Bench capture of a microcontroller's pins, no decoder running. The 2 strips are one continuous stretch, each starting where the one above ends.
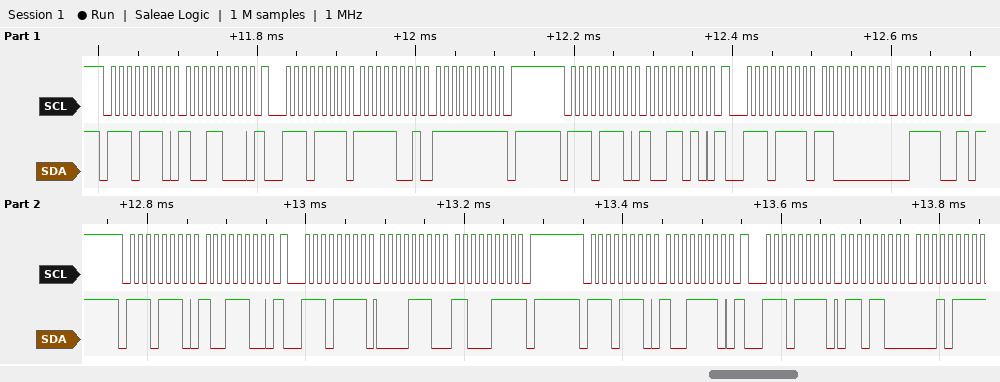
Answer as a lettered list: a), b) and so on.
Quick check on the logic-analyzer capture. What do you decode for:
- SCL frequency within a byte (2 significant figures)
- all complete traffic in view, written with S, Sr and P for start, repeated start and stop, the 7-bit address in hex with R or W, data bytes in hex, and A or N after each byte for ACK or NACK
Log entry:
a) 100 kHz
b) S 77W A 98 A Sr 77R A F9 A FF N P S 77W A 9A A Sr 77R A C0 A 3C N P S 77W A 9C A Sr 77R A 0E A C7 N P S 77W A 9E A Sr 77R A 6C A 17 N
